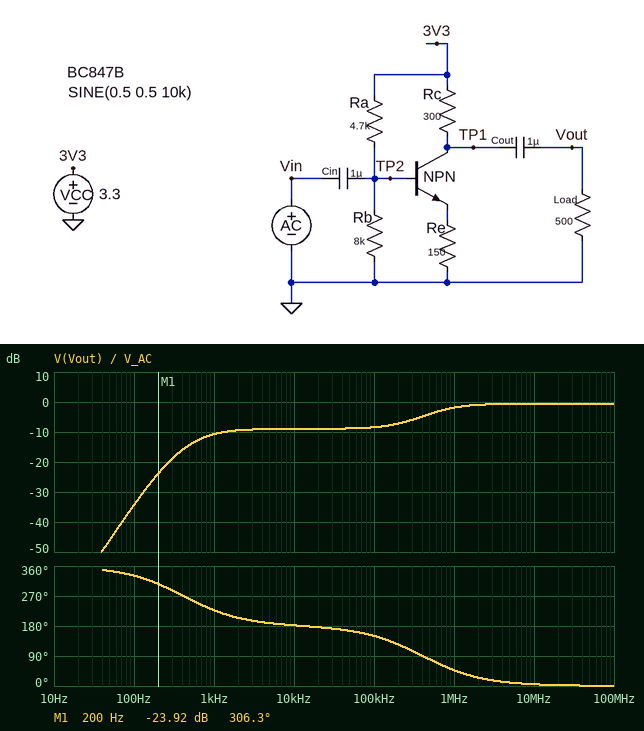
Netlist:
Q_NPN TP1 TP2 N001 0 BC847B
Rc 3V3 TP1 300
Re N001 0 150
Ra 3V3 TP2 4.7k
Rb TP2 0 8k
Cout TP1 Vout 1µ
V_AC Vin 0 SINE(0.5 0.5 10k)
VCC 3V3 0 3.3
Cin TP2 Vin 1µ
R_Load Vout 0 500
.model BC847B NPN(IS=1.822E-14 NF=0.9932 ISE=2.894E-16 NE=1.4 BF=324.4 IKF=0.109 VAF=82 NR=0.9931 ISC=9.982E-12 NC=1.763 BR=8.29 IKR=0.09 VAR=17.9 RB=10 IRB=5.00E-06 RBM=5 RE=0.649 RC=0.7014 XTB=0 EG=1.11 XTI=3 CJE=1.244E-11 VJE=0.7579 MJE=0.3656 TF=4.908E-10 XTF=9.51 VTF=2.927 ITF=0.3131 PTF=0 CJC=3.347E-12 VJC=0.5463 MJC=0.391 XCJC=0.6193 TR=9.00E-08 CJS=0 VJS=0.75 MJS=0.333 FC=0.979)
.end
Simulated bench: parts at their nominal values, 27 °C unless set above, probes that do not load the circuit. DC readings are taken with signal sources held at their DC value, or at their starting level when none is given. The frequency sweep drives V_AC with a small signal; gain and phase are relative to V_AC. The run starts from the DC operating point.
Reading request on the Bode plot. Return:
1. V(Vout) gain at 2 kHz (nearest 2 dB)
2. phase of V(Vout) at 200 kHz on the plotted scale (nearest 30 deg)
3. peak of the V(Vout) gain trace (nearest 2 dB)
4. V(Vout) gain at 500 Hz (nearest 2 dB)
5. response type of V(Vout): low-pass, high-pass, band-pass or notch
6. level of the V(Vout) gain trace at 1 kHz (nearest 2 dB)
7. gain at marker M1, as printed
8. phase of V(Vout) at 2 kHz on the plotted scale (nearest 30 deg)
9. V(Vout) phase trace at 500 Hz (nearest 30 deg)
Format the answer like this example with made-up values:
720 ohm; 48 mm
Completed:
-10 dB; 120 deg; 0 dB; -14 dB; high-pass; -10 dB; -23.92 dB; 210 deg; 270 deg
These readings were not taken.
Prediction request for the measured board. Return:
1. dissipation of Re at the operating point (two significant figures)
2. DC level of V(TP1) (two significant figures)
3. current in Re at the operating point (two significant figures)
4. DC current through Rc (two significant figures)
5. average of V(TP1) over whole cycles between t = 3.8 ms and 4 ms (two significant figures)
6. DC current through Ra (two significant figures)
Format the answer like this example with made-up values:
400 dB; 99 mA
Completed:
7.8 mW; 1.2 V; 7.2 mA; 7.1 mA; 1.7 V; 320 µA
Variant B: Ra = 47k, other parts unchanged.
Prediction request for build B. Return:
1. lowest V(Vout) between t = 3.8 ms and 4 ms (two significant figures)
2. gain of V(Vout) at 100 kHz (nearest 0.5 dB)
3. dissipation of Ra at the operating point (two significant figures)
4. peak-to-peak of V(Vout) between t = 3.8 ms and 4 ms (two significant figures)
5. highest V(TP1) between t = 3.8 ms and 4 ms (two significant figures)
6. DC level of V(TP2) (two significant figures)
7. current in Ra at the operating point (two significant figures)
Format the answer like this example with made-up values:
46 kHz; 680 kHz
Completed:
-290 mV; -35.5 dB; 170 µW; 400 mV; 3.2 V; 480 mV; 60 µA
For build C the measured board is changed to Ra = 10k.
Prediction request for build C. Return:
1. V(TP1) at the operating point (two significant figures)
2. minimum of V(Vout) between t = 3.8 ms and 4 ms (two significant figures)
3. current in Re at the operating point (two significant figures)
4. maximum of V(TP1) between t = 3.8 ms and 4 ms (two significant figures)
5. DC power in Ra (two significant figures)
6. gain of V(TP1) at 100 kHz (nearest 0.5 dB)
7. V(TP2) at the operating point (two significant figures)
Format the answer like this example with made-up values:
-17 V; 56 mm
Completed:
1.9 V; -590 mV; 4.8 mA; 2.5 V; 360 µW; 1.5 dB; 1.4 V
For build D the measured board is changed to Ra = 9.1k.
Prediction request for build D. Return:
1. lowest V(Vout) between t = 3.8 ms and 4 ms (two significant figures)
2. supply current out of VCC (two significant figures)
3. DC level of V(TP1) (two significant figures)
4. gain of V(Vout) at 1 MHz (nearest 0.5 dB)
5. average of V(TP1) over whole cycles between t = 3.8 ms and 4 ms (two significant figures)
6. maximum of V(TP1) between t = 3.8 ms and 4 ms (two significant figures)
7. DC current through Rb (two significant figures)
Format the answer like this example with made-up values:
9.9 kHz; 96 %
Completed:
-560 mV; 5.4 mA; 1.7 V; 1.5 dB; 1.8 V; 2.4 V; 180 µA
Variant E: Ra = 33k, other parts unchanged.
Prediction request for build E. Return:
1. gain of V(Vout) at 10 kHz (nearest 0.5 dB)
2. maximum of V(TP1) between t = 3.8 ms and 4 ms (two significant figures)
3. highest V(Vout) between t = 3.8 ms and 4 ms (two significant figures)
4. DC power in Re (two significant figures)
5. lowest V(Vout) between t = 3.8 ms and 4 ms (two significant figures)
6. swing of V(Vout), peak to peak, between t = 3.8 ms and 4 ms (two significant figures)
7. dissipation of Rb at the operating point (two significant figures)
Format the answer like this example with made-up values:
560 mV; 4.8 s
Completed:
-2.5 dB; 3.2 V; 190 mV; 9.8 µW; -390 mV; 580 mV; 51 µW
